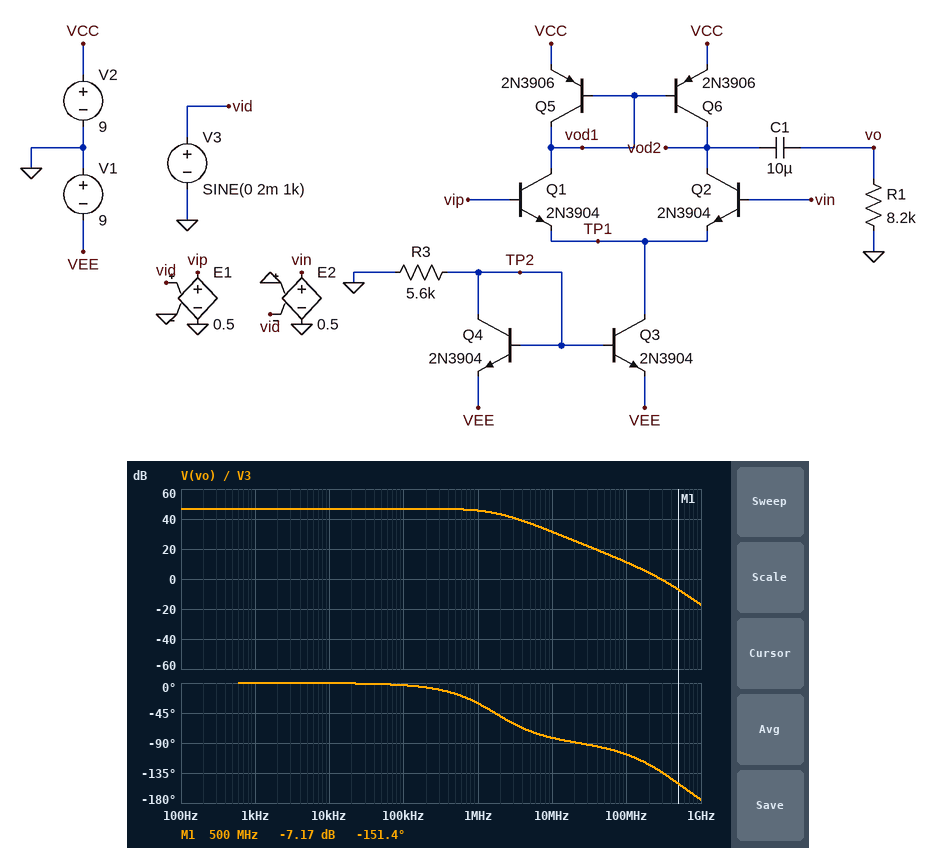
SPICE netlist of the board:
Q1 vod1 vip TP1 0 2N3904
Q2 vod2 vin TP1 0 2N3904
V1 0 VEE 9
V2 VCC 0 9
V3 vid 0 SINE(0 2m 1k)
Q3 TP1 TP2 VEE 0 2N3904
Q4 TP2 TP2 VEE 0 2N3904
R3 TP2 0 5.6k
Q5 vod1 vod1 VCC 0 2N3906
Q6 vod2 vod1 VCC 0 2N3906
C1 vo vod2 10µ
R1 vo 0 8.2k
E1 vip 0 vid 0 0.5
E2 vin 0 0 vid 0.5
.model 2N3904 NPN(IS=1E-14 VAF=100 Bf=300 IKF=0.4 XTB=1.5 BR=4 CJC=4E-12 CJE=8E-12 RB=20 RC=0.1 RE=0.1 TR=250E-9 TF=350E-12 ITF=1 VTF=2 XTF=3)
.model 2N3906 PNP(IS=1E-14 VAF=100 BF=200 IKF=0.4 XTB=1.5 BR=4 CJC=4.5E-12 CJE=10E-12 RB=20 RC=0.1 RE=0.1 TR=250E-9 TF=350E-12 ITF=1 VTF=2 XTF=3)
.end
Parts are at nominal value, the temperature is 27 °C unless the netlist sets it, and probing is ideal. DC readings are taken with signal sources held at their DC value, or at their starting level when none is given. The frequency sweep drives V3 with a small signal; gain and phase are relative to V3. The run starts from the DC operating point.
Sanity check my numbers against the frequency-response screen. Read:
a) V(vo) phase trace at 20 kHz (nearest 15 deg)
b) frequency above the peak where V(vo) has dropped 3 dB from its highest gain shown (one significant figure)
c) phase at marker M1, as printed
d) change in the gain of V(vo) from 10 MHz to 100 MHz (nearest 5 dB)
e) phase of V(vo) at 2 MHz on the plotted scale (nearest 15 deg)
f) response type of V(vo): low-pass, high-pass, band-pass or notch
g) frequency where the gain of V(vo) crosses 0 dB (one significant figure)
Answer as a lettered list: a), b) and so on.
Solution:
a) 0 deg
b) 2 MHz
c) -151.4 deg
d) -20 dB
e) -45 deg
f) low-pass
g) 300 MHz
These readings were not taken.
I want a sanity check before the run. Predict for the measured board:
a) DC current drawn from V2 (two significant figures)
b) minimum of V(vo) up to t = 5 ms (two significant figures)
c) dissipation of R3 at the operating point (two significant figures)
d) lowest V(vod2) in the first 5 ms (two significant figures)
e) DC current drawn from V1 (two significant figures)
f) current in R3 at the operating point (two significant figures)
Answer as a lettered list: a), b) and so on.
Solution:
a) 1.6 mA
b) -440 mV
c) 12 mW
d) 7.4 V
e) 3.1 mA
f) 1.5 mA
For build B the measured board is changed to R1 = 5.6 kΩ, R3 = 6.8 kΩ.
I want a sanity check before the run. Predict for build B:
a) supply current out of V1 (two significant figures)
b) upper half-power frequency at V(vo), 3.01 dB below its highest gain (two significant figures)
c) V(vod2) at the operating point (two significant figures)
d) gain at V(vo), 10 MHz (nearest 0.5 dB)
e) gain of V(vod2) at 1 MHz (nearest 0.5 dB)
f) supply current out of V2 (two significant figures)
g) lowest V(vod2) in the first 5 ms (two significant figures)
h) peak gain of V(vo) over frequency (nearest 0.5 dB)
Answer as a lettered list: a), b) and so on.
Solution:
a) 2.5 mA
b) 2.5 MHz
c) 7.8 V
d) 30.0 dB
e) 41.5 dB
f) 1.3 mA
g) 7.6 V
h) 42.5 dB
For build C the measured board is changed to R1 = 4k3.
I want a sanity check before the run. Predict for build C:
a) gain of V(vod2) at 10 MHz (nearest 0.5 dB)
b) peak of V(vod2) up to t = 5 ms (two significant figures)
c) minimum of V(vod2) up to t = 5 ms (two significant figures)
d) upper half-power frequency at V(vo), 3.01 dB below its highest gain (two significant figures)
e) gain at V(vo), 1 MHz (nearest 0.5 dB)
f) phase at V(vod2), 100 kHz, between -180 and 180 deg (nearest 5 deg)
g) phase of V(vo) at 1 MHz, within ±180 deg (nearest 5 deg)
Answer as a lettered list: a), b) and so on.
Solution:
a) 31.0 dB
b) 8.1 V
c) 7.6 V
d) 3.0 MHz
e) 41.5 dB
f) 0 deg
g) -20 deg
